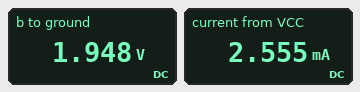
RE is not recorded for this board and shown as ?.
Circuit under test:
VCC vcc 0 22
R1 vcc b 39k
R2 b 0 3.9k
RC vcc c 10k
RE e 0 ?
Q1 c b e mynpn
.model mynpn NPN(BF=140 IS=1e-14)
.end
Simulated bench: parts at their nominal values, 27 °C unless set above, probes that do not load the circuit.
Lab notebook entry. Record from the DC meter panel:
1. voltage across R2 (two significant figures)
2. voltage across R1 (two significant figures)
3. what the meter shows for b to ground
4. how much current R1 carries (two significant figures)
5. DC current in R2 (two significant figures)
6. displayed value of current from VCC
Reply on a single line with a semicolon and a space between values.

1.9 V; 20 V; 1.948 V; 510 µA; 500 µA; 2.555 mA
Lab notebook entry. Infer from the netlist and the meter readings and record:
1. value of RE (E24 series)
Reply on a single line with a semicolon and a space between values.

620 Ω
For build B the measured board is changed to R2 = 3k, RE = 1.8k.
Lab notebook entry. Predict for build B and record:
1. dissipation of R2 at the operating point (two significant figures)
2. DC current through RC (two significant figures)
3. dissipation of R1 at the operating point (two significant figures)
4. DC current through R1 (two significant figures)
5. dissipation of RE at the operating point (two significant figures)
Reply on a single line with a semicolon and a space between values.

810 µW; 510 µA; 11 mW; 520 µA; 470 µW
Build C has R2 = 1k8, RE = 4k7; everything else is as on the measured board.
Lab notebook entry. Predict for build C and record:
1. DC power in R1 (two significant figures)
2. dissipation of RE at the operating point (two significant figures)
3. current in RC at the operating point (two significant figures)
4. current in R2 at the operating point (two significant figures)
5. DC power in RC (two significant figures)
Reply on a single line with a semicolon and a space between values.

11 mW; 31 µW; 80 µA; 540 µA; 64 µW
